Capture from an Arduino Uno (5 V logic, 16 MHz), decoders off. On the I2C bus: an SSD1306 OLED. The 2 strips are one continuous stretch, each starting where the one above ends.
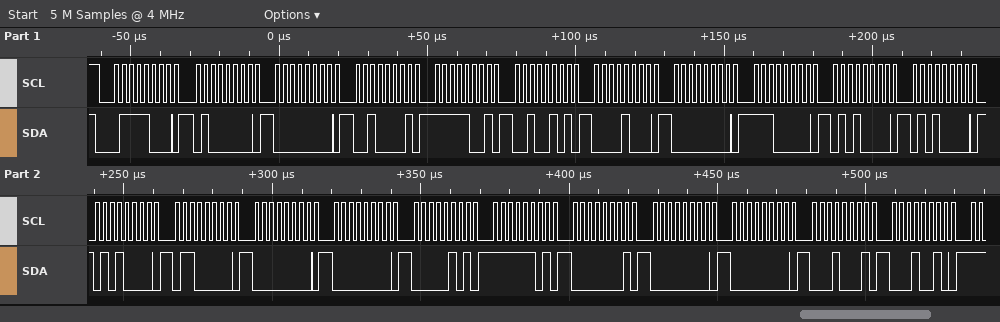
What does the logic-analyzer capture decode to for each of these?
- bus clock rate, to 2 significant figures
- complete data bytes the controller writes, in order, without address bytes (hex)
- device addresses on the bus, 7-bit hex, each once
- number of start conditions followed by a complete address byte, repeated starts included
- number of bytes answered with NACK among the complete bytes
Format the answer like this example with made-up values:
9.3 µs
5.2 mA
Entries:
400 kHz
40 00 21 F9 25 08 00 E0 50 50 50 60 00 00 05 FD 01 00 00 11 12
0x3C
1
0
